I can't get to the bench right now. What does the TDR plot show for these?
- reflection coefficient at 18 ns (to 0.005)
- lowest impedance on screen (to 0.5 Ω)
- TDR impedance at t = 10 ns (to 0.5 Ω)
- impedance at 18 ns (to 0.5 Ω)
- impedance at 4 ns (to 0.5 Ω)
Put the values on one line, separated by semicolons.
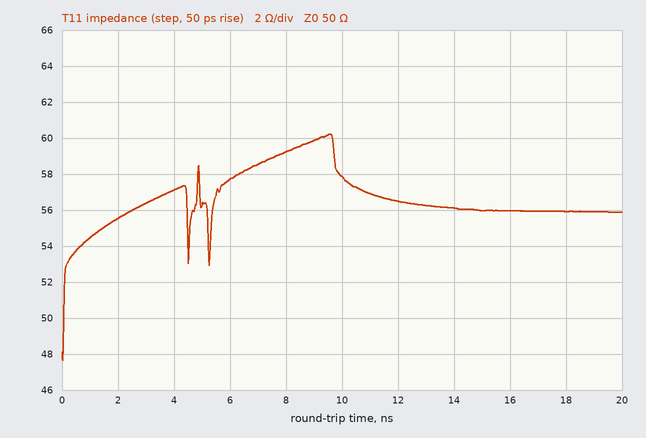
+0.055; 47.5 Ω; 58.0 Ω; 56.0 Ω; 57.0 Ω
